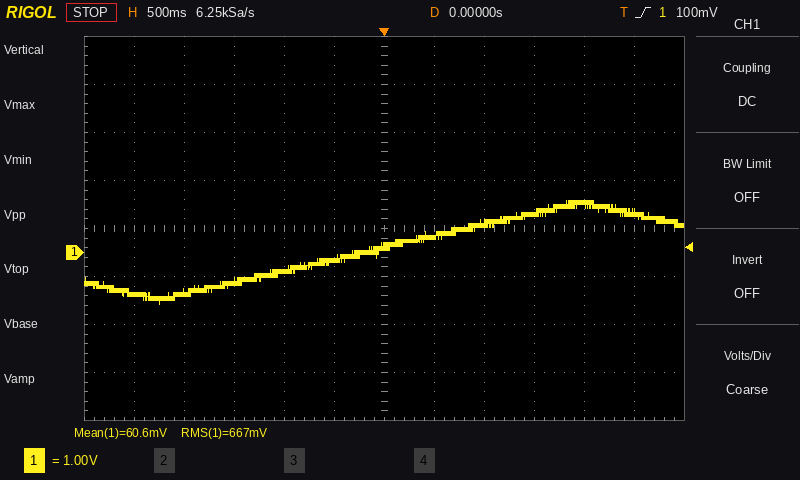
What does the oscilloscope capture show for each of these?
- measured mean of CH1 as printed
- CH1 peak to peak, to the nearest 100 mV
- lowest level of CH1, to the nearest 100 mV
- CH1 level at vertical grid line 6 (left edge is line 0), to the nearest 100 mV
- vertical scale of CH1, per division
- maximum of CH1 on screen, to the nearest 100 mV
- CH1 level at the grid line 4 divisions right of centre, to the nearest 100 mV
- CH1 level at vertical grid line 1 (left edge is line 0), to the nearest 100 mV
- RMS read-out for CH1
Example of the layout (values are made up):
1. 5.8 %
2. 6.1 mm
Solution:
1. 60.6 mV
2. 2.2 V
3. -1.1 V
4. 100 mV
5. 1 V
6. 1.1 V
7. 1.0 V
8. -900 mV
9. 667 mV
